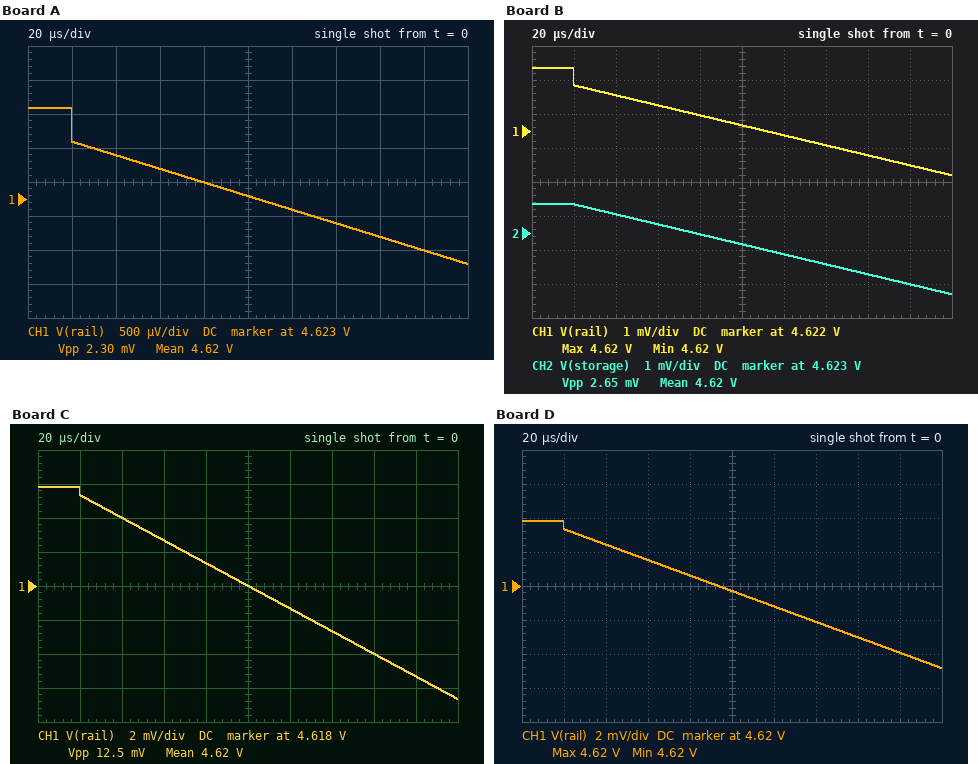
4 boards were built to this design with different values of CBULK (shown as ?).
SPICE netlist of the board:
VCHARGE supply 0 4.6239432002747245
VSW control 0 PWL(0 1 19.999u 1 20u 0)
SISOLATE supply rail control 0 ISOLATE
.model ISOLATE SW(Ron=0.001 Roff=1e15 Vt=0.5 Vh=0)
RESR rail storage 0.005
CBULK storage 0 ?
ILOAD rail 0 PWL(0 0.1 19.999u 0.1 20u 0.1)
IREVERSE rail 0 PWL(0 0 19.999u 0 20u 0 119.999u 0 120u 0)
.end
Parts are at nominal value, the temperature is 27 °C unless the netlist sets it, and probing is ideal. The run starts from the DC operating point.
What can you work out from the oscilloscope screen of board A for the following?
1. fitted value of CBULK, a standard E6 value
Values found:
10 mF
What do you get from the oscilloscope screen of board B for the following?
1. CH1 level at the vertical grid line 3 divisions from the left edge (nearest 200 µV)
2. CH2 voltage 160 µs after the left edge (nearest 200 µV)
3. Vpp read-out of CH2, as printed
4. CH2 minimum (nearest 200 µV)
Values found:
4.6228 V
4.6218 V
2.65 mV
4.6212 V
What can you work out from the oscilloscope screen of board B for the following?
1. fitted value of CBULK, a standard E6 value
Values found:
6.8 mF
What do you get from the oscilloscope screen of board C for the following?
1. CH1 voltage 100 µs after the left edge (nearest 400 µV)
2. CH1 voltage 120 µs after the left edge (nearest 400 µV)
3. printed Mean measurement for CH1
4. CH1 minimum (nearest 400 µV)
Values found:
4.6180 V
4.6168 V
4.62 V
4.6112 V
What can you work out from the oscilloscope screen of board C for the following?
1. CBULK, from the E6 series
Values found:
1.5 mF
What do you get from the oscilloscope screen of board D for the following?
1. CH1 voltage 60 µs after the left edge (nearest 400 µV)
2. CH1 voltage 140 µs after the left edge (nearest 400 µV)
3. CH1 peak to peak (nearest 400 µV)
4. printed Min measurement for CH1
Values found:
4.6216 V
4.6180 V
8.8 mV
4.62 V
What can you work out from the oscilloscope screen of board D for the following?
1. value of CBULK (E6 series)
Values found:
2.2 mF
